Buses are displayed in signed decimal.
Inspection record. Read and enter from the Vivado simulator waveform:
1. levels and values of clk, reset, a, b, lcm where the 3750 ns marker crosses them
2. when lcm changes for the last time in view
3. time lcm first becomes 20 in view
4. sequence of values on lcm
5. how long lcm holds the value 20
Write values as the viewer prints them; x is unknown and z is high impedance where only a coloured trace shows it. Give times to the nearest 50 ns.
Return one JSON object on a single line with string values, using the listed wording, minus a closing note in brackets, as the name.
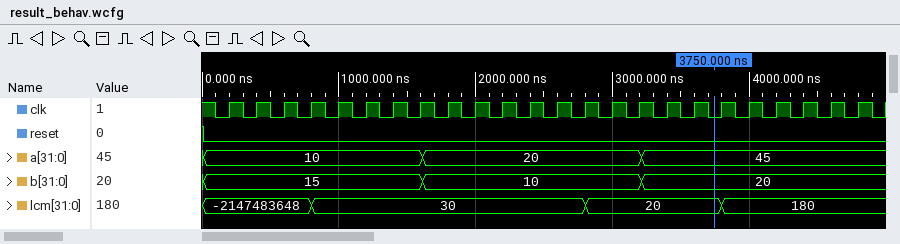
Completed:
{"levels and values of clk, reset, a, b, lcm where the 3750 ns marker crosses them": "clk=0, reset=0, a=45, b=20, lcm=20", "when lcm changes for the last time in view": "3800 ns", "time lcm first becomes 20 in view": "2800 ns", "sequence of values on lcm": "-2147483648, 30, 20, 180", "how long lcm holds the value 20": "1000 ns"}
